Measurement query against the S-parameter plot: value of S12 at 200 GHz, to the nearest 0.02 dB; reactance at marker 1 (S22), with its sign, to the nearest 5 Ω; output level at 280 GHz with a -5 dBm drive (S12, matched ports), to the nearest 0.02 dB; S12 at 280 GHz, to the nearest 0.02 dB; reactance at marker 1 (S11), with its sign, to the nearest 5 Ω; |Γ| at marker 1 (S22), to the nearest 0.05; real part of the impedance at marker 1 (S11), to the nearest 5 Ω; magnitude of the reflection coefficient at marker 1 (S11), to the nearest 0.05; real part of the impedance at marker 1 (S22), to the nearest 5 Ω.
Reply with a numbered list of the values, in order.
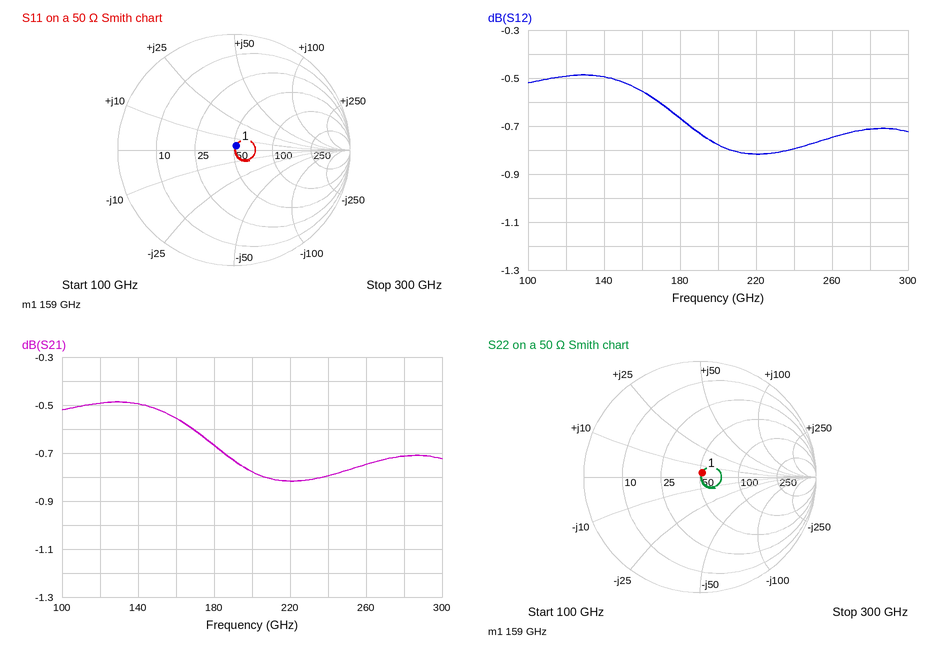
1. -0.78 dB
2. +5 Ω
3. -5.72 dBm
4. -0.72 dB
5. +5 Ω
6. 0.05
7. 50 Ω
8. 0.05
9. 50 Ω
